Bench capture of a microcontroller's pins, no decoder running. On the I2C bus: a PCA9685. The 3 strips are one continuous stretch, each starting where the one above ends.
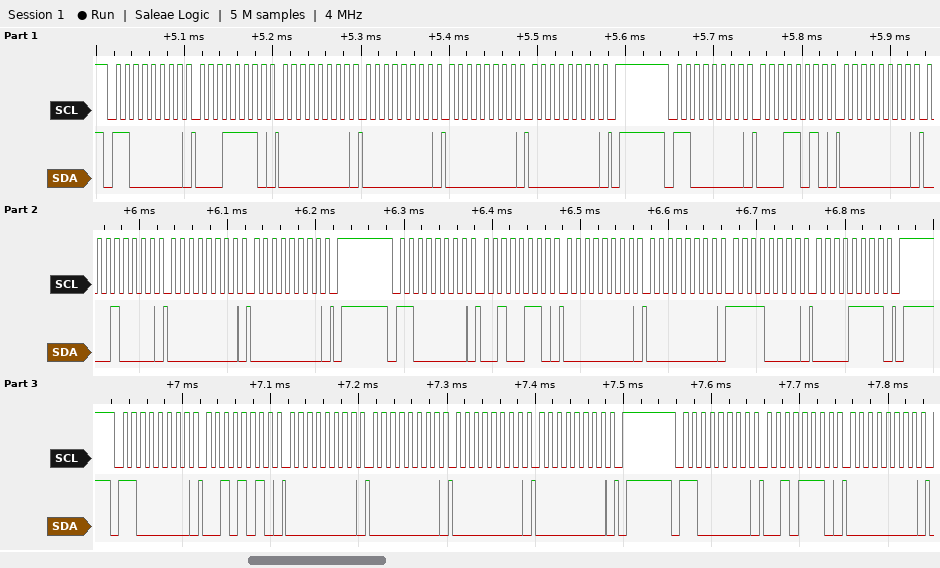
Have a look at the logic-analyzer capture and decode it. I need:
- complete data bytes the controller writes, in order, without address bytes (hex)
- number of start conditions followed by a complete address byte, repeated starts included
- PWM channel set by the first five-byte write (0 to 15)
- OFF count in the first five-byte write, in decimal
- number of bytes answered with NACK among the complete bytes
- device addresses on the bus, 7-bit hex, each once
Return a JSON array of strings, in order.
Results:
["1E 00 00 00 00 1A 00 10 00 00 26 00 00 F0 0F 2A 00 00 00 00 2E 00", "5", "6", "0", "0", "0x60"]
